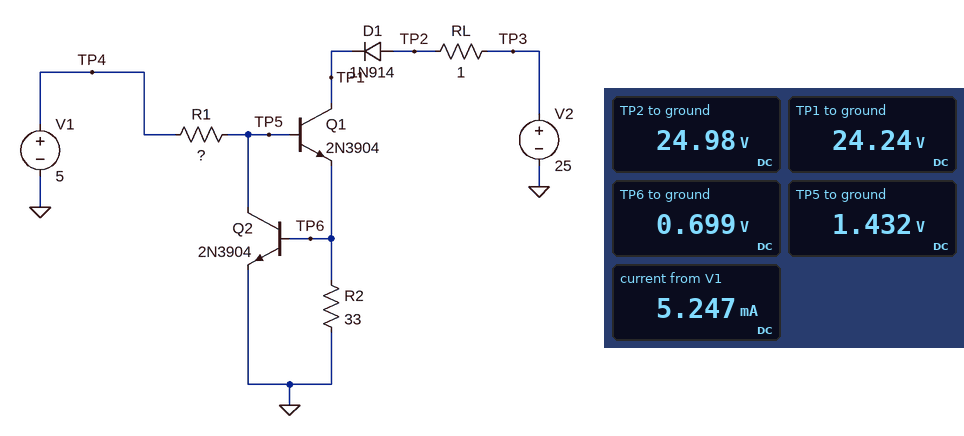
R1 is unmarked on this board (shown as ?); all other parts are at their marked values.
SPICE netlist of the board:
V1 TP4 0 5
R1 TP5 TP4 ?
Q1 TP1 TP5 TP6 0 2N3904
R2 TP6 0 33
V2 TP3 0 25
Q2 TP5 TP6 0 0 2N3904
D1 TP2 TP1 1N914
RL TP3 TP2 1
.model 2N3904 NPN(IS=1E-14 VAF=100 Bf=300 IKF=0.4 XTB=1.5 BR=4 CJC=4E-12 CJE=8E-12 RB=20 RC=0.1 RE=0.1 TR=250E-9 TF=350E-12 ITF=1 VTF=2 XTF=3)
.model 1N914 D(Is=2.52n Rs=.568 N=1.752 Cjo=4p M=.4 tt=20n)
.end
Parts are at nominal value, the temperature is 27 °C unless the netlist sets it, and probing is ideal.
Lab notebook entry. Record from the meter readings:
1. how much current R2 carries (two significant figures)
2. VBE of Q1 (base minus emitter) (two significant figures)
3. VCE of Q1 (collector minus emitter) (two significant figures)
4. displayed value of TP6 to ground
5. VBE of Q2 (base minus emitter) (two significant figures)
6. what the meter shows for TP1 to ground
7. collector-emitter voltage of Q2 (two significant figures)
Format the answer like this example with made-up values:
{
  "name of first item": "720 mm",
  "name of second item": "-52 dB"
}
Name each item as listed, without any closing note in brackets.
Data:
{
  "how much current R2 carries": "21 mA",
  "VBE of Q1 (base minus emitter)": "730 mV",
  "VCE of Q1 (collector minus emitter)": "24 V",
  "displayed value of TP6 to ground": "0.699 V",
  "VBE of Q2 (base minus emitter)": "700 mV",
  "what the meter shows for TP1 to ground": "24.24 V",
  "collector-emitter voltage of Q2": "1.4 V"
}
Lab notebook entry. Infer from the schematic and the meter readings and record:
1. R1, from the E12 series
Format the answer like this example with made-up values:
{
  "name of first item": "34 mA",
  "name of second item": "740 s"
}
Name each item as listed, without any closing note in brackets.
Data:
{
  "R1, from the E12 series": "680 Ω"
}
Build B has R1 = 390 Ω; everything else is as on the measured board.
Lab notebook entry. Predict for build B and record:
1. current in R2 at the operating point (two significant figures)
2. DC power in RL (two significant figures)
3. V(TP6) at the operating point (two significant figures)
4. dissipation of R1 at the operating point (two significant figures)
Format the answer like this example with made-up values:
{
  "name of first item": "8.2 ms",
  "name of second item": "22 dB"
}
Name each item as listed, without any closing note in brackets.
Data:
{
  "current in R2 at the operating point": "22 mA",
  "DC power in RL": "470 µW",
  "V(TP6) at the operating point": "710 mV",
  "dissipation of R1 at the operating point": "32 mW"
}
